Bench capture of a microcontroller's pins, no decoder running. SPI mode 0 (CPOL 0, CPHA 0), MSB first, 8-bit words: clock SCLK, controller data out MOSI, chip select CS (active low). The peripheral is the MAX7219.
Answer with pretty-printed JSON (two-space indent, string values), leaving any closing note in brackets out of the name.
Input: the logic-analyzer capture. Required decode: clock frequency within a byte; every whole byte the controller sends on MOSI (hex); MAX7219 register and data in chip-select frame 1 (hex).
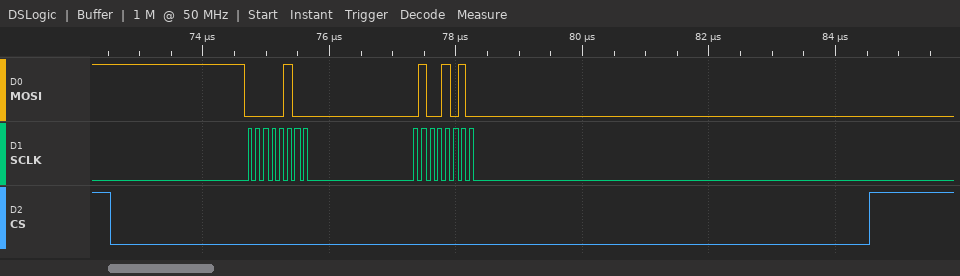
{
  "clock frequency within a byte": "8 MHz",
  "every whole byte the controller sends on MOSI": "04 4A",
  "MAX7219 register and data in chip-select frame 1": "register 0x4, data 0x4A"
}
